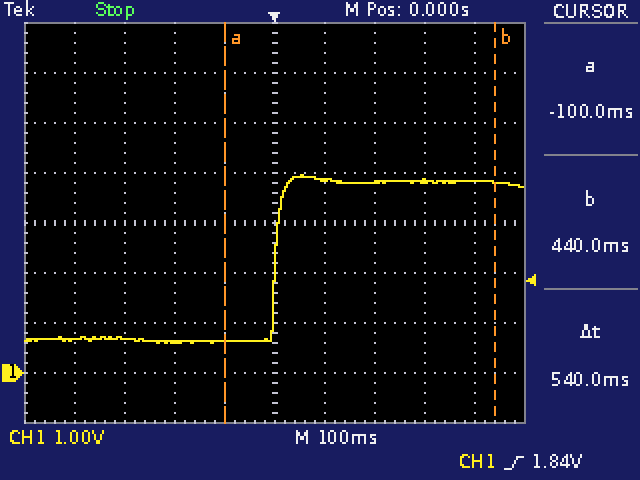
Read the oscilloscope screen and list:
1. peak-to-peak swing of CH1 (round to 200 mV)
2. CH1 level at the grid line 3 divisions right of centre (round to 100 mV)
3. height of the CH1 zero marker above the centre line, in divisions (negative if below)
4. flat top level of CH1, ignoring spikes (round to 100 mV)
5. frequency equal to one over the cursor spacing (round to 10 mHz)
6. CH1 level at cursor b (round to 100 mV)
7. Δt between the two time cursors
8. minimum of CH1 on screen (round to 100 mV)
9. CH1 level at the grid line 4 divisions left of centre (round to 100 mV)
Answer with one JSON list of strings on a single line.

["3.4 V", "3.8 V", "-3.0 div", "3.8 V", "1.85 Hz", "3.8 V", "540 ms", "600 mV", "700 mV"]
